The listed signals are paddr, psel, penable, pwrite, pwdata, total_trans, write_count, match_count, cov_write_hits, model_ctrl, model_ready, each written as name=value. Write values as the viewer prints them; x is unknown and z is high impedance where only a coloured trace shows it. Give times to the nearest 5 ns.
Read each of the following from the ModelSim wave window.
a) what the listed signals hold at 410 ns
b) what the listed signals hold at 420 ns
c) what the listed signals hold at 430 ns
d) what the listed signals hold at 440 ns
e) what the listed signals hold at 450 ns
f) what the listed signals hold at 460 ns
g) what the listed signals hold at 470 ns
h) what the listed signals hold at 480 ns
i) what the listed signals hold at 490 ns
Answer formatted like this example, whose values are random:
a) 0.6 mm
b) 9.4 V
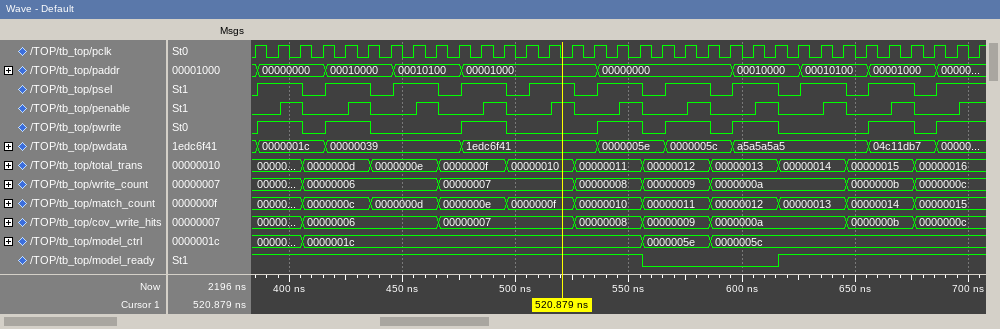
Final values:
a) paddr=00000000, psel=0, penable=0, pwrite=0, pwdata=0000001c, total_trans=0000000d, write_count=00000006, match_count=0000000c, cov_write_hits=00000006, model_ctrl=0000001c, model_ready=1
b) paddr=00010000, psel=1, penable=0, pwrite=1, pwdata=00000039, total_trans=0000000d, write_count=00000006, match_count=0000000c, cov_write_hits=00000006, model_ctrl=0000001c, model_ready=1
c) paddr=00010000, psel=1, penable=1, pwrite=1, pwdata=00000039, total_trans=0000000d, write_count=00000006, match_count=0000000c, cov_write_hits=00000006, model_ctrl=0000001c, model_ready=1
d) paddr=00010000, psel=0, penable=0, pwrite=0, pwdata=00000039, total_trans=0000000e, write_count=00000006, match_count=0000000d, cov_write_hits=00000006, model_ctrl=0000001c, model_ready=1
e) paddr=00010100, psel=1, penable=0, pwrite=0, pwdata=00000039, total_trans=0000000e, write_count=00000006, match_count=0000000d, cov_write_hits=00000006, model_ctrl=0000001c, model_ready=1
f) paddr=00010100, psel=1, penable=1, pwrite=0, pwdata=00000039, total_trans=0000000e, write_count=00000006, match_count=0000000d, cov_write_hits=00000006, model_ctrl=0000001c, model_ready=1
g) paddr=00010100, psel=0, penable=0, pwrite=0, pwdata=00000039, total_trans=0000000f, write_count=00000007, match_count=0000000e, cov_write_hits=00000007, model_ctrl=0000001c, model_ready=1
h) paddr=00001000, psel=1, penable=0, pwrite=1, pwdata=1edc6f41, total_trans=0000000f, write_count=00000007, match_count=0000000e, cov_write_hits=00000007, model_ctrl=0000001c, model_ready=1
i) paddr=00001000, psel=1, penable=1, pwrite=1, pwdata=1edc6f41, total_trans=0000000f, write_count=00000007, match_count=0000000e, cov_write_hits=00000007, model_ctrl=0000001c, model_ready=1
